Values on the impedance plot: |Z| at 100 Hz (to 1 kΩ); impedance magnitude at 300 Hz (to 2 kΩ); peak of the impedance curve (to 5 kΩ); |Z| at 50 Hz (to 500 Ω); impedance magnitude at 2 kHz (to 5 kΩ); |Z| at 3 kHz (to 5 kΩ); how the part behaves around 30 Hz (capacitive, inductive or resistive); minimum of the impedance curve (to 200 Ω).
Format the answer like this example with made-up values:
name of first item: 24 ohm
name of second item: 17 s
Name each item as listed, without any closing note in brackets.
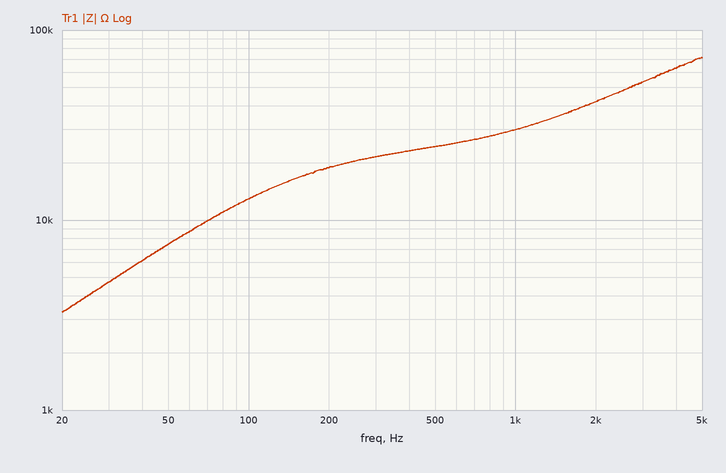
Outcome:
|Z| at 100 Hz: 13 kΩ
impedance magnitude at 300 Hz: 22 kΩ
peak of the impedance curve: 70 kΩ
|Z| at 50 Hz: 7.5 kΩ
impedance magnitude at 2 kHz: 40 kΩ
|Z| at 3 kHz: 55 kΩ
how the part behaves around 30 Hz: inductive
minimum of the impedance curve: 3.2 kΩ
